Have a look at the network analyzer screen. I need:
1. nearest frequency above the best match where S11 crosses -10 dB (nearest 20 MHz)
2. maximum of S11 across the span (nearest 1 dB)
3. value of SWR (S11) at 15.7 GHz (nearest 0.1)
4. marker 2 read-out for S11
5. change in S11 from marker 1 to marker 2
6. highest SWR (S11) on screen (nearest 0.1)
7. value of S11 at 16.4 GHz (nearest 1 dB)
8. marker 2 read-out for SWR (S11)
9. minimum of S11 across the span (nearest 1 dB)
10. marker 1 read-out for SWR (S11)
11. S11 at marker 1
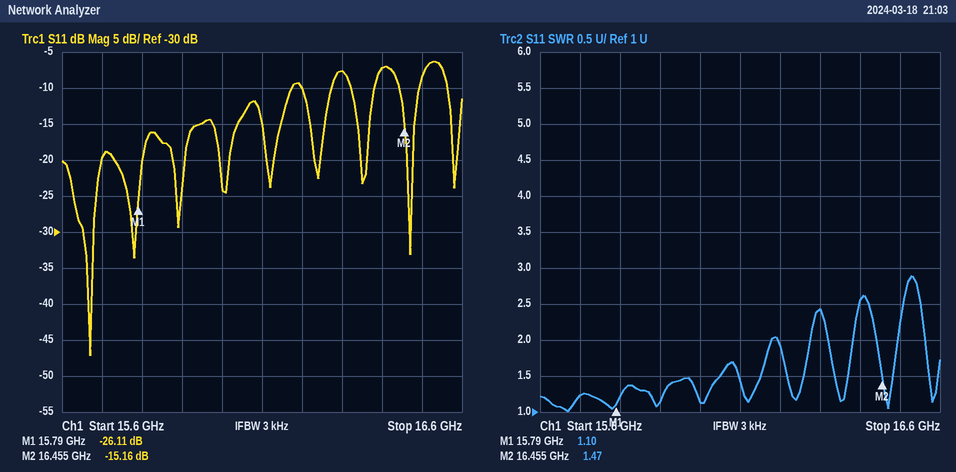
16.18 GHz
-6 dB
1.2
-15.16 dB
10.95 dB
2.9
-7 dB
1.47
-47 dB
1.10
-26.11 dB
